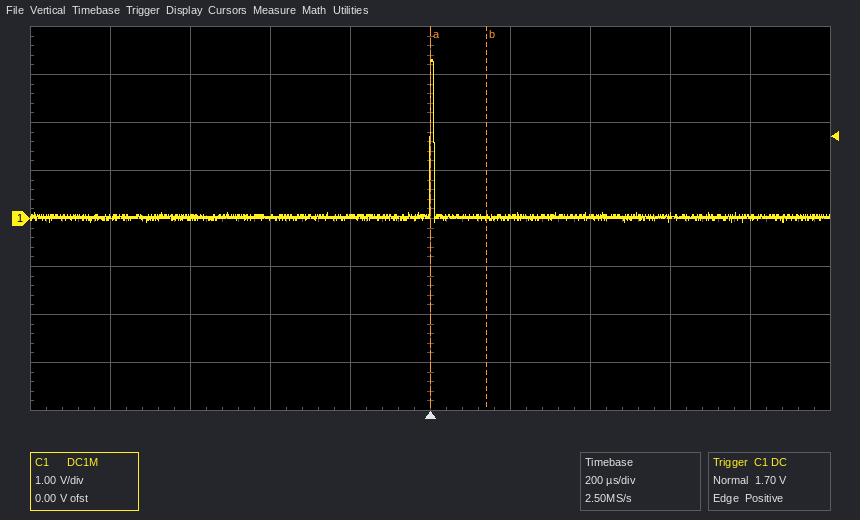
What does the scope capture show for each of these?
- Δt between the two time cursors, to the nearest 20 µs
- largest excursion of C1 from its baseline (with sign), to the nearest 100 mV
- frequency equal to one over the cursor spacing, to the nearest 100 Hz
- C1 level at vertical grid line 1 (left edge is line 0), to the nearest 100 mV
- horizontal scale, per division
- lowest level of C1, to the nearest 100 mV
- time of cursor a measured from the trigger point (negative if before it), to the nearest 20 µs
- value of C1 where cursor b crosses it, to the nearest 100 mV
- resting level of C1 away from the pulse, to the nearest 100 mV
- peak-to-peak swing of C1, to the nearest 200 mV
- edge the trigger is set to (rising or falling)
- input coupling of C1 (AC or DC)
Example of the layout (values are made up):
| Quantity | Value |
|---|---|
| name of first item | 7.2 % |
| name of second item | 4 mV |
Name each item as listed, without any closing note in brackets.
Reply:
| Quantity | Value |
|---|---|
| Δt between the two time cursors, to the nearest 20 µs | 140 µs |
| largest excursion of C1 from its baseline (with sign), to the nearest 100 mV | +3.3 V |
| frequency equal to one over the cursor spacing, to the nearest 100 Hz | 7.1 kHz |
| C1 level at vertical grid line 1 (left edge is line 0), to the nearest 100 mV | 0.0 V |
| horizontal scale, per division | 200 µs |
| lowest level of C1, to the nearest 100 mV | -100 mV |
| time of cursor a measured from the trigger point (negative if before it), to the nearest 20 µs | 0 µs |
| value of C1 where cursor b crosses it, to the nearest 100 mV | 0.0 V |
| resting level of C1 away from the pulse, to the nearest 100 mV | 0.0 V |
| peak-to-peak swing of C1, to the nearest 200 mV | 3.4 V |
| edge the trigger is set to | rising |
| input coupling of C1 | DC |
